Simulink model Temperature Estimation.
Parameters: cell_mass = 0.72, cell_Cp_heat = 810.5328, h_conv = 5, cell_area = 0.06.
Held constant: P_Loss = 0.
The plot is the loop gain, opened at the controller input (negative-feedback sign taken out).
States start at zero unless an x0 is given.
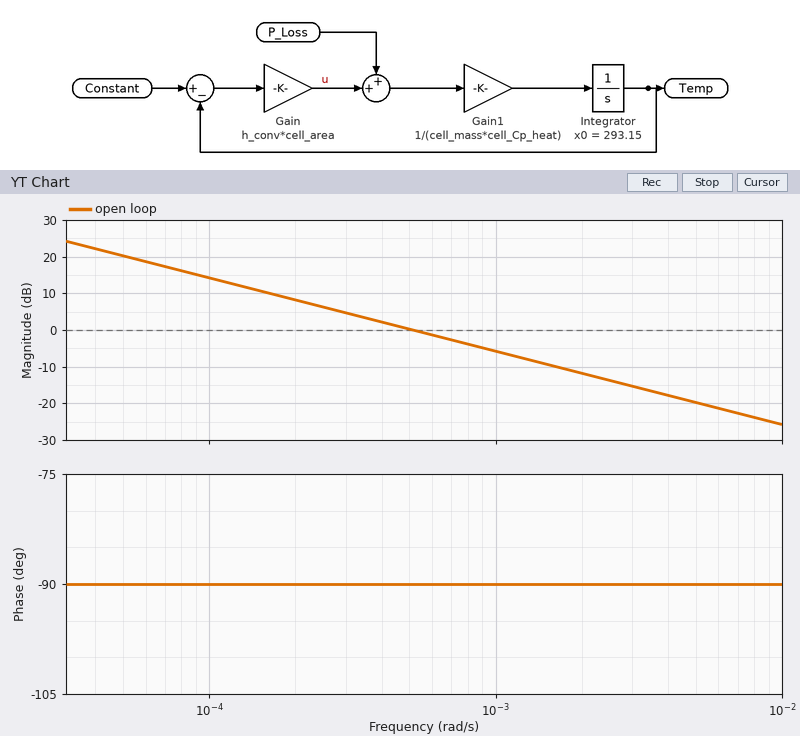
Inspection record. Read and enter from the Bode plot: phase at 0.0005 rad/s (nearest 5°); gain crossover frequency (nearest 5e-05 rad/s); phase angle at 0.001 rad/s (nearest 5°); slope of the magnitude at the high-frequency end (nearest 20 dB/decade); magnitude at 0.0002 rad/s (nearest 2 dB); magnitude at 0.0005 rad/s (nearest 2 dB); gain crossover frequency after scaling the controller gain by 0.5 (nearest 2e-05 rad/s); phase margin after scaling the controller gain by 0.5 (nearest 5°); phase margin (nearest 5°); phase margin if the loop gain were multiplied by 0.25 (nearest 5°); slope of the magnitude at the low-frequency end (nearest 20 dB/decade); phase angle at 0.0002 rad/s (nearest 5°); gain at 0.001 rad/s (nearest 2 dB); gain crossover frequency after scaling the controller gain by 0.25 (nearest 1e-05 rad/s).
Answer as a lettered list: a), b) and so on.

a) -90°
b) 0.00050 rad/s
c) -90°
d) -20 dB/decade
e) 8 dB
f) 0 dB
g) 0.00026 rad/s
h) 90°
i) 90°
j) 90°
k) -20 dB/decade
l) -90°
m) -6 dB
n) 0.00013 rad/s
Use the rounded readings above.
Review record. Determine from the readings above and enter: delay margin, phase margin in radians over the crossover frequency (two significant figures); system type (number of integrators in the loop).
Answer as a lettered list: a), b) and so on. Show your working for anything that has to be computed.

a) 90 × π / 180 / 0.0005 = 3100 s
b) 1
